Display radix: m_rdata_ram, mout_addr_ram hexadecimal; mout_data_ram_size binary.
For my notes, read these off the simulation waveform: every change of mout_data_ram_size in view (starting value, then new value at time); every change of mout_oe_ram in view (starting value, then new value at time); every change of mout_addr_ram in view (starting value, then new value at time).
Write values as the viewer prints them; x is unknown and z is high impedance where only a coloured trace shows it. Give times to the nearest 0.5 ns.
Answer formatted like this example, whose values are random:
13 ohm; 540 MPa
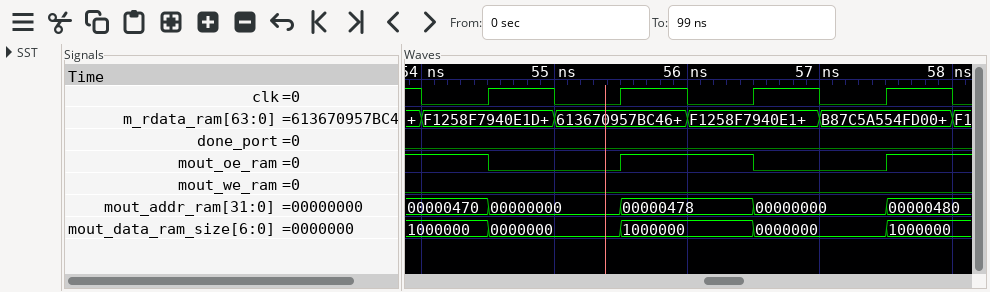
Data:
1000000, 0000000 at 54.5 ns, 1000000 at 55.5 ns, 0000000 at 56.5 ns, 1000000 at 57.5 ns; 1, 0 at 54.5 ns, 1 at 55.5 ns, 0 at 56.5 ns, 1 at 57.5 ns; 00000470, 00000000 at 54.5 ns, 00000478 at 55.5 ns, 00000000 at 56.5 ns, 00000480 at 57.5 ns
